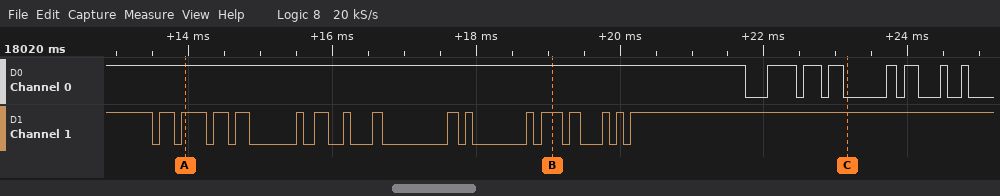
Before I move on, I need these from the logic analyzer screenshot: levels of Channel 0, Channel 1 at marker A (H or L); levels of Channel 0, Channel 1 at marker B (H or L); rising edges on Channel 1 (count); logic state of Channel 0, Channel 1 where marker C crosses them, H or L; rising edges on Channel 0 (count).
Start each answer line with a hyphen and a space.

- Channel 0=H, Channel 1=H
- Channel 0=H, Channel 1=H
- 16
- Channel 0=L, Channel 1=H
- 7
